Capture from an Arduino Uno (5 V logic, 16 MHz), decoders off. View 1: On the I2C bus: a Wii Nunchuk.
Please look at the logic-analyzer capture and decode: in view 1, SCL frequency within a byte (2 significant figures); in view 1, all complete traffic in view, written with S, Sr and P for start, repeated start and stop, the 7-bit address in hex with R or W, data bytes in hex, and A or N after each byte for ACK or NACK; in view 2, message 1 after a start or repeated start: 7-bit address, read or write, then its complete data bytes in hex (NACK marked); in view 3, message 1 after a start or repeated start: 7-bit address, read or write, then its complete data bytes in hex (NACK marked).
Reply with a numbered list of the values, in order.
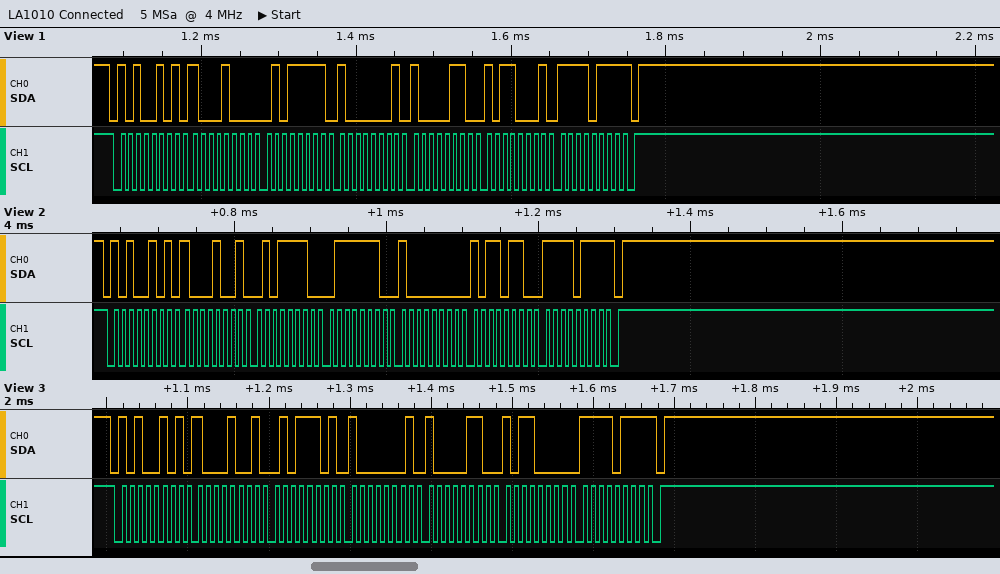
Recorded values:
1. 100 kHz
2. S 52R A 88 A 5F A 81 A 86 A B1 A F7 N P
3. 0x52 read: 89 5E 7E 80 B6 F7 NACK
4. 0x52 read: 89 5D 81 86 B0 F7 NACK
